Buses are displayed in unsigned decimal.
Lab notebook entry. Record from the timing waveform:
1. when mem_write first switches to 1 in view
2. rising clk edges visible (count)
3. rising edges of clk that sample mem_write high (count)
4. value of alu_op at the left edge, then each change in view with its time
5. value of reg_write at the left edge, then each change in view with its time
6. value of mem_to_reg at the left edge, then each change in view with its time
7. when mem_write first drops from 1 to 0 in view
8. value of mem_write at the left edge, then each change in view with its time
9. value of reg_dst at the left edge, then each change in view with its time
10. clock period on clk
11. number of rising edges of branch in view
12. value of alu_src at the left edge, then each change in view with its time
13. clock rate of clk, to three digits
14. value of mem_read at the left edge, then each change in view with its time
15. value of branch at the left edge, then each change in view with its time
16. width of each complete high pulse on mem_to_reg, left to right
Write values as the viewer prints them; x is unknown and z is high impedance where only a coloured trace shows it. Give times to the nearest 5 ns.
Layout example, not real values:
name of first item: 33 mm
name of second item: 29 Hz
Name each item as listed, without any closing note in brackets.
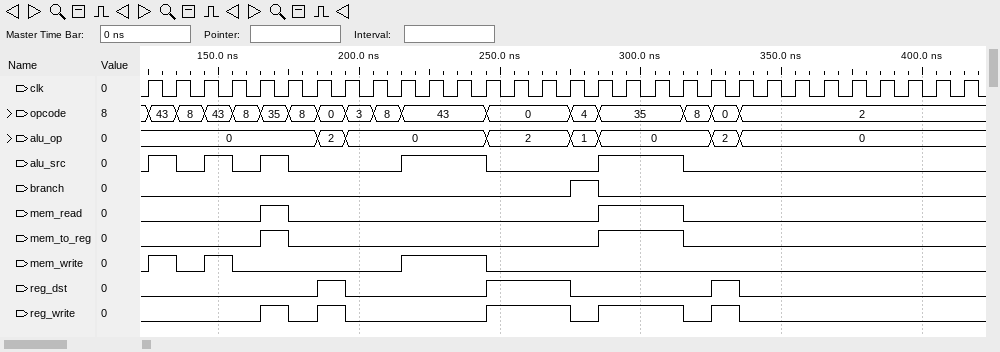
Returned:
when mem_write first switches to 1 in view: 125 ns
rising clk edges visible: 30
rising edges of clk that sample mem_write high: 5
value of alu_op at the left edge, then each change in view with its time: 0, 2 at 185 ns, 0 at 195 ns, 2 at 245 ns, 1 at 275 ns, 0 at 285 ns, 2 at 325 ns, 0 at 335 ns
value of reg_write at the left edge, then each change in view with its time: 0, 1 at 165 ns, 0 at 175 ns, 1 at 185 ns, 0 at 195 ns, 1 at 245 ns, 0 at 275 ns, 1 at 285 ns, 0 at 315 ns, 1 at 325 ns, 0 at 335 ns
value of mem_to_reg at the left edge, then each change in view with its time: 0, 1 at 165 ns, 0 at 175 ns, 1 at 285 ns, 0 at 315 ns
when mem_write first drops from 1 to 0 in view: 135 ns
value of mem_write at the left edge, then each change in view with its time: 0, 1 at 125 ns, 0 at 135 ns, 1 at 145 ns, 0 at 155 ns, 1 at 215 ns, 0 at 245 ns
value of reg_dst at the left edge, then each change in view with its time: 0, 1 at 185 ns, 0 at 195 ns, 1 at 245 ns, 0 at 275 ns, 1 at 325 ns, 0 at 335 ns
clock period on clk: 10 ns
number of rising edges of branch in view: 1
value of alu_src at the left edge, then each change in view with its time: 0, 1 at 125 ns, 0 at 135 ns, 1 at 145 ns, 0 at 155 ns, 1 at 165 ns, 0 at 175 ns, 1 at 215 ns, 0 at 245 ns, 1 at 285 ns, 0 at 315 ns
clock rate of clk, to three digits: 100 MHz
value of mem_read at the left edge, then each change in view with its time: 0, 1 at 165 ns, 0 at 175 ns, 1 at 285 ns, 0 at 315 ns
value of branch at the left edge, then each change in view with its time: 0, 1 at 275 ns, 0 at 285 ns
width of each complete high pulse on mem_to_reg, left to right: 10 ns, 30 ns
